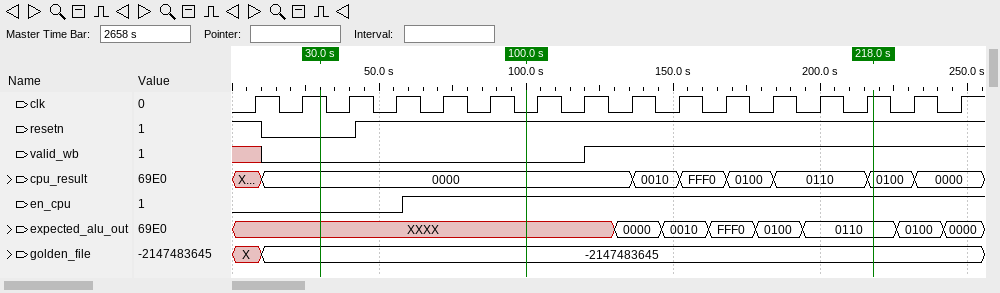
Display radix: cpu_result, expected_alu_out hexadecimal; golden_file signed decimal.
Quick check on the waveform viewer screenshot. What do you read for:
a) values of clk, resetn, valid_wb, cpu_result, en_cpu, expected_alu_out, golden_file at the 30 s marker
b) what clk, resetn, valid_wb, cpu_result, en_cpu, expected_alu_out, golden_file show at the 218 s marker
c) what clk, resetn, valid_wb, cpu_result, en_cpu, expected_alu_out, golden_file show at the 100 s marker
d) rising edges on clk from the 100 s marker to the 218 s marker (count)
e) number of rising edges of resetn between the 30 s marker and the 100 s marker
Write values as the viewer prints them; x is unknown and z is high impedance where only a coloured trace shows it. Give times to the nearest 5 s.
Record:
clk=1, resetn=0, valid_wb=0, cpu_result=0000, en_cpu=0, expected_alu_out=XXXX, golden_file=-2147483645
clk=1, resetn=1, valid_wb=1, cpu_result=0100, en_cpu=1, expected_alu_out=0110, golden_file=-2147483645
clk=0, resetn=1, valid_wb=0, cpu_result=0000, en_cpu=1, expected_alu_out=XXXX, golden_file=-2147483645
8
1
